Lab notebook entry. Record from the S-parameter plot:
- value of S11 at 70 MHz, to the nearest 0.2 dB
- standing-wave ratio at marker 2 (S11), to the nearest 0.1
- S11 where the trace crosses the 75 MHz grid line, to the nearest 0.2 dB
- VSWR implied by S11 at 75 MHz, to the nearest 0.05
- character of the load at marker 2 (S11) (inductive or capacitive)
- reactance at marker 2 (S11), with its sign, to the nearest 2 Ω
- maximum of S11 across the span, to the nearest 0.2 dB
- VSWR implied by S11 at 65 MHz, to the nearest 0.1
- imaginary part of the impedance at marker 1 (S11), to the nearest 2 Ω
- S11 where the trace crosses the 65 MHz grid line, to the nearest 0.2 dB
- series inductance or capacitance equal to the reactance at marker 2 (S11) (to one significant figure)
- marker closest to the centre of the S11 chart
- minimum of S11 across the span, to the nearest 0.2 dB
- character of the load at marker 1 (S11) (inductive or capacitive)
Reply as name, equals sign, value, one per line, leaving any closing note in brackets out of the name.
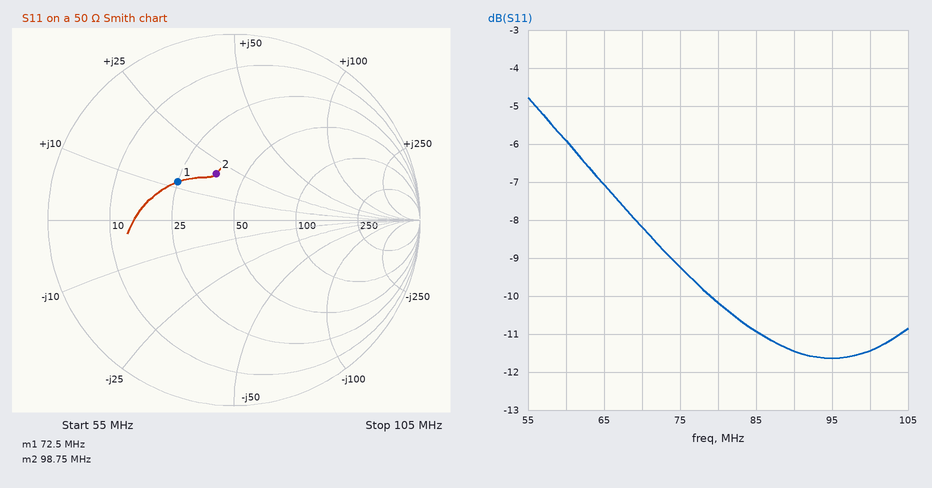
value of S11 at 70 MHz, to the nearest 0.2 dB = -8.2 dB
standing-wave ratio at marker 2 (S11), to the nearest 0.1 = 1.7
S11 where the trace crosses the 75 MHz grid line, to the nearest 0.2 dB = -9.2 dB
VSWR implied by S11 at 75 MHz, to the nearest 0.05 = 2.05
character of the load at marker 2 (S11) = inductive
reactance at marker 2 (S11), with its sign, to the nearest 2 Ω = +20 Ω
maximum of S11 across the span, to the nearest 0.2 dB = -4.8 dB
VSWR implied by S11 at 65 MHz, to the nearest 0.1 = 2.6
imaginary part of the impedance at marker 1 (S11), to the nearest 2 Ω = +12 Ω
S11 where the trace crosses the 65 MHz grid line, to the nearest 0.2 dB = -7.0 dB
series inductance or capacitance equal to the reactance at marker 2 (S11) = 30 nH
marker closest to the centre of the S11 chart = marker 2
minimum of S11 across the span, to the nearest 0.2 dB = -11.6 dB
character of the load at marker 1 (S11) = inductive
